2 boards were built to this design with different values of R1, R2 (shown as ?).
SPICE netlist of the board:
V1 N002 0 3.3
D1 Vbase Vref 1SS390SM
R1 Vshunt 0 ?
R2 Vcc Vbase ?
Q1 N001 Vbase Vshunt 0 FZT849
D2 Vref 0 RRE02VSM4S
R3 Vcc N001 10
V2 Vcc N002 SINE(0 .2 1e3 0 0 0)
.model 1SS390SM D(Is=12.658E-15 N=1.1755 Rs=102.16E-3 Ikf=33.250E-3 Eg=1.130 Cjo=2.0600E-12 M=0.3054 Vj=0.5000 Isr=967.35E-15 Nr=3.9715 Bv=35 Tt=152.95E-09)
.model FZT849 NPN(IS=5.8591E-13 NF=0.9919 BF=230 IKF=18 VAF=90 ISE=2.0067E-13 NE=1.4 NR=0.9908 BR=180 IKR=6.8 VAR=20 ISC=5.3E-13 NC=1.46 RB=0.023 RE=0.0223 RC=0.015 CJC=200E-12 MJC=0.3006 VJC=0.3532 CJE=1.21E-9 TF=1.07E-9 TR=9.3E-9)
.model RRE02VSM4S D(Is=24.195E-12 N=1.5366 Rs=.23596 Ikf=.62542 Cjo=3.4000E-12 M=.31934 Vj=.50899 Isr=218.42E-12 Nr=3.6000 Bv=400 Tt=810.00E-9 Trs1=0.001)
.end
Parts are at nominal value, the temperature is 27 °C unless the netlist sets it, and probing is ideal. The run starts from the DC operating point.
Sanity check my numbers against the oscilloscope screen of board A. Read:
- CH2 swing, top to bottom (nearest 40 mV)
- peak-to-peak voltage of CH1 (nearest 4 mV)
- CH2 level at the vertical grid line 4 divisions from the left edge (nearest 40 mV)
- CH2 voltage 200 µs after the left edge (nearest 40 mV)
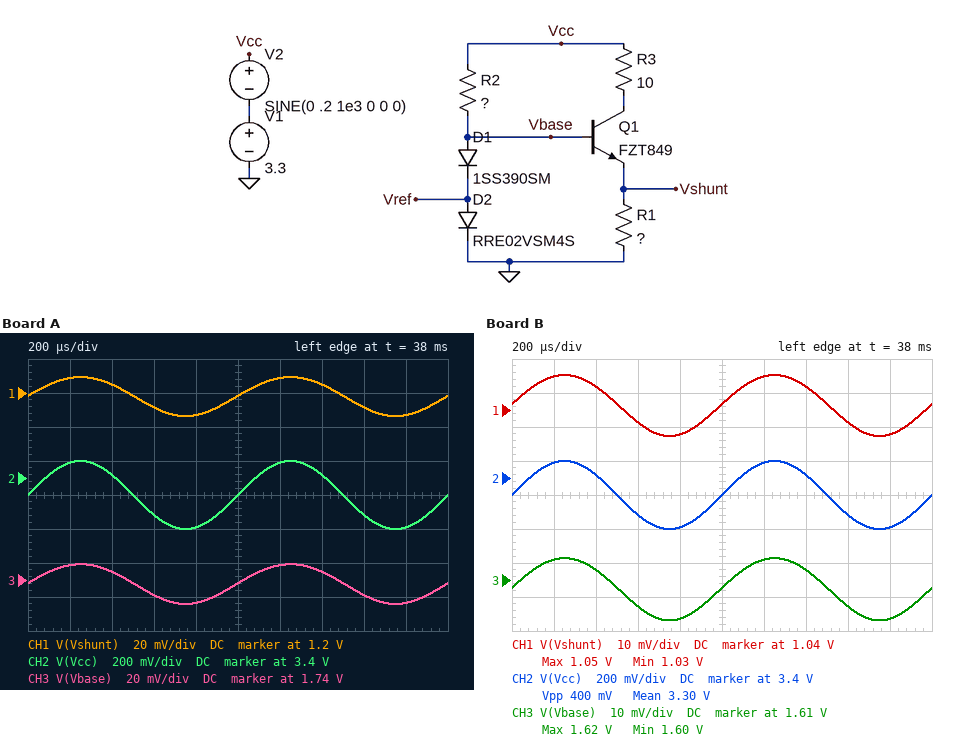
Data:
400 mV
24 mV
3.12 V
3.48 V
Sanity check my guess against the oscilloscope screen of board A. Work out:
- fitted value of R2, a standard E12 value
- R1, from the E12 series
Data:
56 Ω
1.5 kΩ
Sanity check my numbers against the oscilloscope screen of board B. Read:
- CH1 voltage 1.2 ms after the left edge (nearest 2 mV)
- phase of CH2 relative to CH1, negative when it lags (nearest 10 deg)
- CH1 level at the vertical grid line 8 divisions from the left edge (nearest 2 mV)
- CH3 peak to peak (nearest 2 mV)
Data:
1.050 V
0 deg
1.036 V
18 mV
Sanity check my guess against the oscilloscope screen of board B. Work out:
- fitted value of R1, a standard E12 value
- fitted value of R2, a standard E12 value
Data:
470 Ω
270 Ω
